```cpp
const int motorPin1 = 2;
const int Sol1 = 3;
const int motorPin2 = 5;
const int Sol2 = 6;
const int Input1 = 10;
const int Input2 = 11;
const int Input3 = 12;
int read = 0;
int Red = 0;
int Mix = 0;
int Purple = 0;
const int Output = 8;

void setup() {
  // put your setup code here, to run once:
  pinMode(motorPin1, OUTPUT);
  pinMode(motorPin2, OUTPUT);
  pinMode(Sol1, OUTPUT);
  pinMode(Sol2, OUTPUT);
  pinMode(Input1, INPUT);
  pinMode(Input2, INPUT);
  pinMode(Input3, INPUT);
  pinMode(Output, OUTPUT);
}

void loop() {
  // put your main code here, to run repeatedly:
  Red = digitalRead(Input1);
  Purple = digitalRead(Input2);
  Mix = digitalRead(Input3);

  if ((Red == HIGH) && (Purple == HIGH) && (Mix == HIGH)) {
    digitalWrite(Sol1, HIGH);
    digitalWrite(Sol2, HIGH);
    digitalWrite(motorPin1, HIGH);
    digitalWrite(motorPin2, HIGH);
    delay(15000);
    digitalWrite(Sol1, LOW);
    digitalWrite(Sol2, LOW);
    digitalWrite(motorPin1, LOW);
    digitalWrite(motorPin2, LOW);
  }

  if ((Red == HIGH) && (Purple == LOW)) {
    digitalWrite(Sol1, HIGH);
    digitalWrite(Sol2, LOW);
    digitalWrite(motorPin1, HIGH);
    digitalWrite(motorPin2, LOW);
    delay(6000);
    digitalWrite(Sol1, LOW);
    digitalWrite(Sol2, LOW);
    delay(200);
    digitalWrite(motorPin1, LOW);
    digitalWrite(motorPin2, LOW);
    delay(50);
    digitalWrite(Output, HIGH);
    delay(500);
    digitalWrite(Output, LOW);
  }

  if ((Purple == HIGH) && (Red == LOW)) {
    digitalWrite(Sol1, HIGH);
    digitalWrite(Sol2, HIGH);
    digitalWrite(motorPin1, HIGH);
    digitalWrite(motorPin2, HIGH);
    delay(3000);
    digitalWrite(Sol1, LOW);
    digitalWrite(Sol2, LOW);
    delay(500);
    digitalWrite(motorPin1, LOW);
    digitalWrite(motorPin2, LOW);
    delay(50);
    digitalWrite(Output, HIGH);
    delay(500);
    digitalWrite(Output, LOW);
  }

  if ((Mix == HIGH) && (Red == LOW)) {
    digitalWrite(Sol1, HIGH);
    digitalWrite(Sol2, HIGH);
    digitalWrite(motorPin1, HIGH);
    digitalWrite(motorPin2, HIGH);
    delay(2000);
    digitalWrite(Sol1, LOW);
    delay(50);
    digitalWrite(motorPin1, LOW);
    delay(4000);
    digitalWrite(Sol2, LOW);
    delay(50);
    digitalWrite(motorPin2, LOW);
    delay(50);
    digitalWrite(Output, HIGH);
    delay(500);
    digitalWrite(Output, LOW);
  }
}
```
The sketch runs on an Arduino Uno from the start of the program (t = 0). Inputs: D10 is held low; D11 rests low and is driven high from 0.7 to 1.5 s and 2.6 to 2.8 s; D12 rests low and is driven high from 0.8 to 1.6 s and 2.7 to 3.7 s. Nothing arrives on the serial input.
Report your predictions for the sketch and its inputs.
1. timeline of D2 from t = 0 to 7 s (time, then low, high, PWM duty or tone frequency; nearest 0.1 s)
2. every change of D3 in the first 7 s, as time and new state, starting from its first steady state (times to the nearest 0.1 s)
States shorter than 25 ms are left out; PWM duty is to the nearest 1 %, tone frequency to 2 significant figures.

0 s low; 0.7 s high; 4.2 s low
0 s low; 0.7 s high; 3.7 s low
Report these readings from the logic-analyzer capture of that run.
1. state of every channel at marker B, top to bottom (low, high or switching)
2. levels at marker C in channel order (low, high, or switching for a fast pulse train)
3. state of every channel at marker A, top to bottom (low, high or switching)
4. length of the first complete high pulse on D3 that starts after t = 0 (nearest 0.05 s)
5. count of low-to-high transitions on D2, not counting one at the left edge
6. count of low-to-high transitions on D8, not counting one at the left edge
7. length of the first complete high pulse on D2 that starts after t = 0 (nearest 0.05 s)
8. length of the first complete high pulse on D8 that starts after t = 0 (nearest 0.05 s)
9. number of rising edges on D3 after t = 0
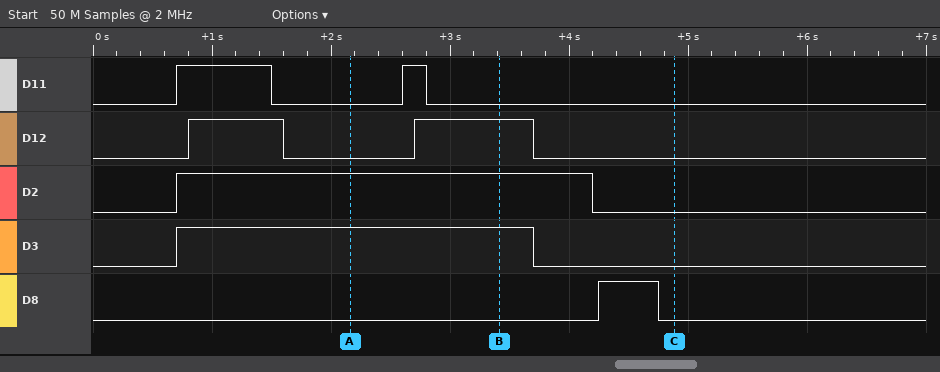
D11 low, D12 high, D2 high, D3 high, D8 low
D11 low, D12 low, D2 low, D3 low, D8 low
D11 low, D12 low, D2 high, D3 high, D8 low
3.00 s
1
1
3.50 s
0.50 s
1
